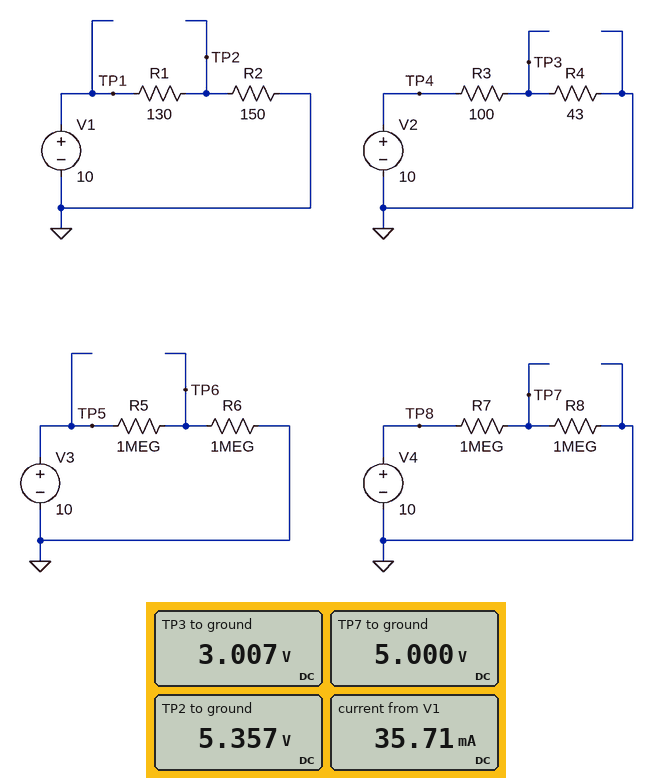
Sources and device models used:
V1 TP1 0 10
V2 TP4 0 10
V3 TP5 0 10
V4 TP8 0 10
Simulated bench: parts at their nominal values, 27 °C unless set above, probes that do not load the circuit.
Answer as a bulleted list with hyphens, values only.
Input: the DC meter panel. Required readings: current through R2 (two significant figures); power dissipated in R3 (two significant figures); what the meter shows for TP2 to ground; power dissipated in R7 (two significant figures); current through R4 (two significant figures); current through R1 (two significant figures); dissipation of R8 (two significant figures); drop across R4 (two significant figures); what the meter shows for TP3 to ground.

- 36 mA
- 490 mW
- 5.357 V
- 25 µW
- 70 mA
- 36 mA
- 25 µW
- 3.0 V
- 3.007 V
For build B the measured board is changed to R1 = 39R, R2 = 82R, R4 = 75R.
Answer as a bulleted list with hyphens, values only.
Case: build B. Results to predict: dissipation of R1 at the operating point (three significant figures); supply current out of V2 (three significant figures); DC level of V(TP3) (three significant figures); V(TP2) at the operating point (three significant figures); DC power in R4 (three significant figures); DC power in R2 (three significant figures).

- 266 mW
- 57.1 mA
- 4.29 V
- 6.78 V
- 245 mW
- 560 mW
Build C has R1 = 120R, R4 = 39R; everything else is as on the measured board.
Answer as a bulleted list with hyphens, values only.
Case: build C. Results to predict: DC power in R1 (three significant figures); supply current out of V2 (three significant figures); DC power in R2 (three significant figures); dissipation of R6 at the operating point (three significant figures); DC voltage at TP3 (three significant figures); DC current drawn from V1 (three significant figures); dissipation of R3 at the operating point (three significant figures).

- 165 mW
- 71.9 mA
- 206 mW
- 25.0 µW
- 2.81 V
- 37.0 mA
- 518 mW
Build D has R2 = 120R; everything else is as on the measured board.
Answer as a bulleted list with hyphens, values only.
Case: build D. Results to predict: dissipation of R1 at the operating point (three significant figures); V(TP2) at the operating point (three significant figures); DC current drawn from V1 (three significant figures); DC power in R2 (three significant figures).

- 208 mW
- 4.80 V
- 40.0 mA
- 192 mW
